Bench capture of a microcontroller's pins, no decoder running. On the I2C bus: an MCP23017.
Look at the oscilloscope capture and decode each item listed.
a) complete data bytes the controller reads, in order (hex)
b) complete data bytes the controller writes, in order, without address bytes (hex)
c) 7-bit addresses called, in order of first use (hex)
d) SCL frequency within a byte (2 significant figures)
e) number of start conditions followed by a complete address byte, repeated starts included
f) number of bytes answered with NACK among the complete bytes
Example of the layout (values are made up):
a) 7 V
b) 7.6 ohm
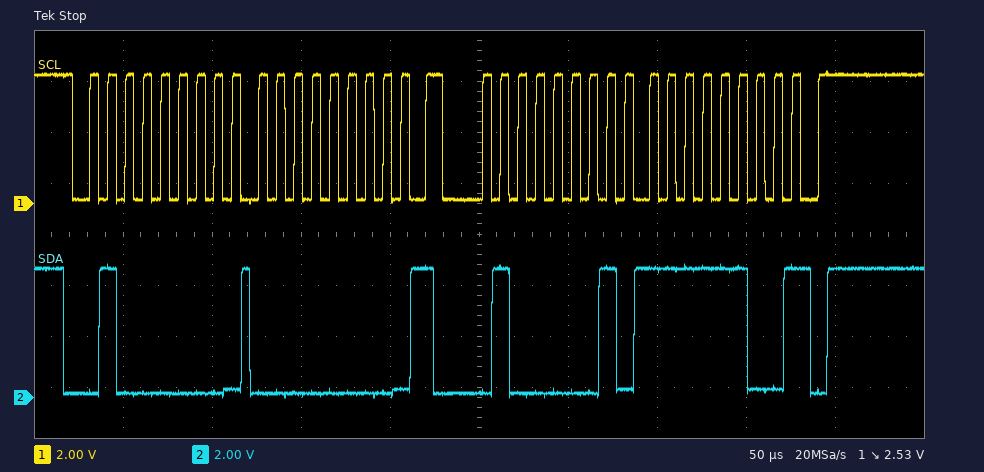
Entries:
a) FC
b) 00
c) 0x20
d) 100 kHz
e) 2
f) 1
